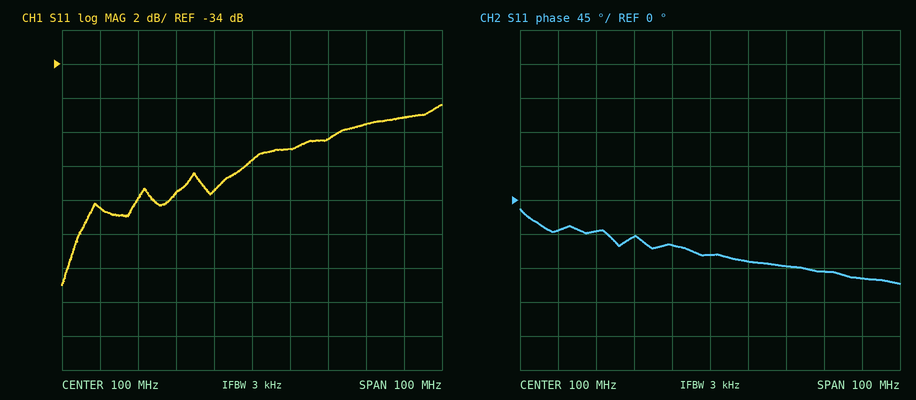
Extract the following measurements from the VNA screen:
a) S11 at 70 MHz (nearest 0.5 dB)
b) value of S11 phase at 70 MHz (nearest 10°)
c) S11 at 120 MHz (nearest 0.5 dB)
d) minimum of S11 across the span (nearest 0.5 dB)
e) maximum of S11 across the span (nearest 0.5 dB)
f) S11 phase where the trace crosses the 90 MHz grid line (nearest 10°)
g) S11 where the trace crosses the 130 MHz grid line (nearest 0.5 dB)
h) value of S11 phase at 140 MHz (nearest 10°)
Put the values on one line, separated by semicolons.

-42.0 dB; -40°; -38.5 dB; -47.0 dB; -36.5 dB; -60°; -37.5 dB; -100°
